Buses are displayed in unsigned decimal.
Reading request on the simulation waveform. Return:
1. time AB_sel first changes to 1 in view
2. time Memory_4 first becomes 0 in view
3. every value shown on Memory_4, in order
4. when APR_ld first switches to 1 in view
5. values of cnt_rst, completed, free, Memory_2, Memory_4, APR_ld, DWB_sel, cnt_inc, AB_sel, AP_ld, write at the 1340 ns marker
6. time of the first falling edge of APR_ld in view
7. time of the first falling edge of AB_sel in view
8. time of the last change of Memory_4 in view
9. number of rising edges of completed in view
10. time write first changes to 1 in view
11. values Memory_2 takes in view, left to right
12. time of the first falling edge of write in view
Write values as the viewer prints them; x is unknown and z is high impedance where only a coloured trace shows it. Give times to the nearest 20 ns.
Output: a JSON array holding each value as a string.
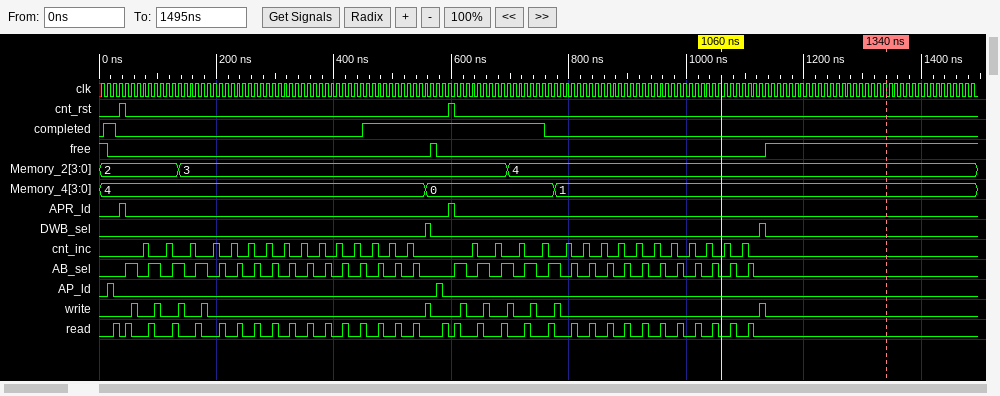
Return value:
["40 ns", "560 ns", "4, 0, 1", "40 ns", "cnt_rst=0, completed=0, free=1, Memory_2=4, Memory_4=1, APR_ld=0, DWB_sel=0, cnt_inc=0, AB_sel=0, AP_ld=0, write=0", "40 ns", "60 ns", "780 ns", "2", "60 ns", "2, 3, 4", "60 ns"]
